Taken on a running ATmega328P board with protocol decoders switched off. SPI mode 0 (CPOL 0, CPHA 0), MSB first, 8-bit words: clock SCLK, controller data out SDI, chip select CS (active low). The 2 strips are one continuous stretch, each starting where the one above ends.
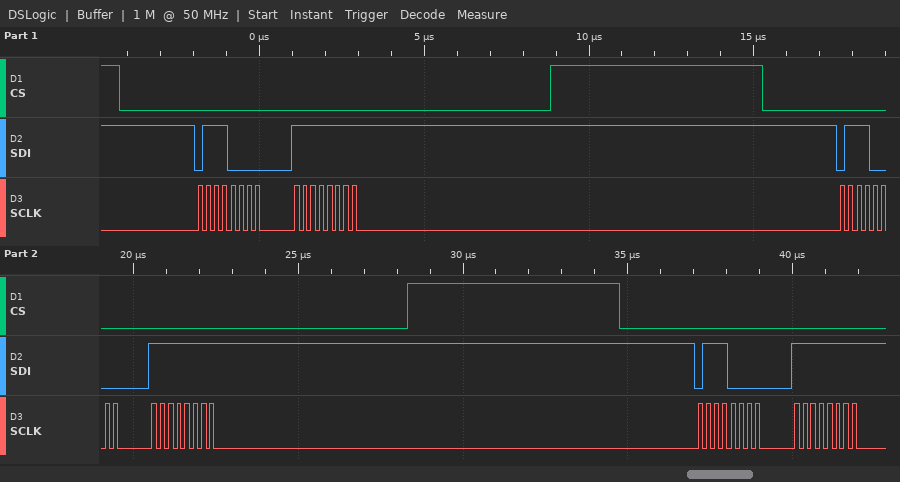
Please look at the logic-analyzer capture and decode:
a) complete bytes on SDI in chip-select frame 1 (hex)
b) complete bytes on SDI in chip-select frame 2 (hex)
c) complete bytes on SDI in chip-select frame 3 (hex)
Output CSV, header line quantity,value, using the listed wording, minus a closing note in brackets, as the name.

quantity,value
complete bytes on SDI in chip-select frame 1,70 FF
complete bytes on SDI in chip-select frame 2,70 FF
complete bytes on SDI in chip-select frame 3,70 FF
